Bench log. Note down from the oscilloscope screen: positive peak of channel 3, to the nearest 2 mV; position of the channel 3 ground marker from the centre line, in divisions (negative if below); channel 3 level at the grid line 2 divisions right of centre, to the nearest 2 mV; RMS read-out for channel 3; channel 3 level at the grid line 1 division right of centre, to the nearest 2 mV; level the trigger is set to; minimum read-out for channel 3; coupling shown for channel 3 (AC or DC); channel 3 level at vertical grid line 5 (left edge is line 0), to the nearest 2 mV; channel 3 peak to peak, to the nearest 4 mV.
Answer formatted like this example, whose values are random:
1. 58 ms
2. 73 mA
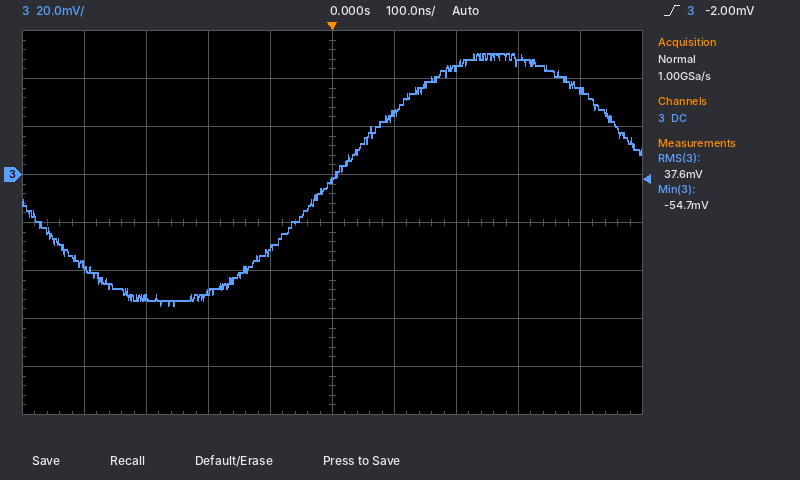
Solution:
1. 50 mV
2. +1.0 div
3. 44 mV
4. 37.6 mV
5. 26 mV
6. -2.00 mV
7. -54.7 mV
8. DC
9. -2 mV
10. 104 mV
